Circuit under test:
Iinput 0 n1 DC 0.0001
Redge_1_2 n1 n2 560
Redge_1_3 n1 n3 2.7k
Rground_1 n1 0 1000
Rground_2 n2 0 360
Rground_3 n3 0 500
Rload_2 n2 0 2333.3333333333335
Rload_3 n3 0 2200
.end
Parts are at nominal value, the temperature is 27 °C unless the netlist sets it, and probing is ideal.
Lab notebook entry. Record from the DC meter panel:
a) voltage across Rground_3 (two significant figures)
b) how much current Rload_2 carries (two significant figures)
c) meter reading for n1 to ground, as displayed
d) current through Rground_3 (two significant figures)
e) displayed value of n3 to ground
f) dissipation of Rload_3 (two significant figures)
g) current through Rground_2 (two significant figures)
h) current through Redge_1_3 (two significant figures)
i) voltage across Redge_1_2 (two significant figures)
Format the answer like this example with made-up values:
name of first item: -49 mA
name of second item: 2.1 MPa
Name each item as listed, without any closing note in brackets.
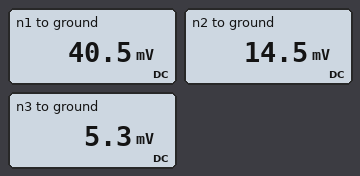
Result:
voltage across Rground_3: 5.3 mV
how much current Rload_2 carries: 6.2 µA
meter reading for n1 to ground, as displayed: 40.5 mV
current through Rground_3: 11 µA
displayed value of n3 to ground: 5.3 mV
dissipation of Rload_3: 13 nW
current through Rground_2: 40 µA
current through Redge_1_3: 13 µA
voltage across Redge_1_2: 26 mV
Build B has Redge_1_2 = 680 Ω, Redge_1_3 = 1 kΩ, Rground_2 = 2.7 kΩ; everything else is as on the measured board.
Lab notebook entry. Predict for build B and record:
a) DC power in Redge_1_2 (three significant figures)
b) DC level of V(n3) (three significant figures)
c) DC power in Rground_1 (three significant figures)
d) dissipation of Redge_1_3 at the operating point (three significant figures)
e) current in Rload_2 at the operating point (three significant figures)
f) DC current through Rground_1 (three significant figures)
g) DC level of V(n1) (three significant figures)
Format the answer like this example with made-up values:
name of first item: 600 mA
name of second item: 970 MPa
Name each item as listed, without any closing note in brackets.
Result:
DC power in Redge_1_2: 367 nW
DC level of V(n3): 13.0 mV
DC power in Rground_1: 2.01 µW
dissipation of Redge_1_3 at the operating point: 1.02 µW
current in Rload_2 at the operating point: 12.5 µA
DC current through Rground_1: 44.9 µA
DC level of V(n1): 44.9 mV
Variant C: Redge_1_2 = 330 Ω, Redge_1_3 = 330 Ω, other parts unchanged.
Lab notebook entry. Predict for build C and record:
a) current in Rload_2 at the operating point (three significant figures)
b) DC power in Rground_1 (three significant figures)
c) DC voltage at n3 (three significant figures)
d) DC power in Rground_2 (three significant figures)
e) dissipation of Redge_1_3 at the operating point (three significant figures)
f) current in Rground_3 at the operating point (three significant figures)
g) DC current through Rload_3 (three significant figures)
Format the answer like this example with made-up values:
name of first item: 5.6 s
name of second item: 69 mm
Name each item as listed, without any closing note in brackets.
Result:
current in Rload_2 at the operating point: 5.32 µA
DC power in Rground_1: 653 nW
DC voltage at n3: 14.1 mV
DC power in Rground_2: 428 nW
dissipation of Redge_1_3 at the operating point: 396 nW
current in Rground_3 at the operating point: 28.2 µA
DC current through Rload_3: 6.42 µA
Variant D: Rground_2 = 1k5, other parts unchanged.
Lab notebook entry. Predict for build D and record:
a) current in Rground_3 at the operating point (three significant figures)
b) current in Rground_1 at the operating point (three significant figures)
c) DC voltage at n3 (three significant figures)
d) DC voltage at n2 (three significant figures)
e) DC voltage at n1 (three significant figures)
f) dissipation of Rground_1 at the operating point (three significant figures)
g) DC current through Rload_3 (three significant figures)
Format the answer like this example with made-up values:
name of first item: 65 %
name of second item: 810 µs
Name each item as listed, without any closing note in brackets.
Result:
current in Rground_3 at the operating point: 13.1 µA
current in Rground_1 at the operating point: 50.0 µA
DC voltage at n3: 6.55 mV
DC voltage at n2: 31.0 mV
DC voltage at n1: 50.0 mV
dissipation of Rground_1 at the operating point: 2.50 µW
DC current through Rload_3: 2.98 µA
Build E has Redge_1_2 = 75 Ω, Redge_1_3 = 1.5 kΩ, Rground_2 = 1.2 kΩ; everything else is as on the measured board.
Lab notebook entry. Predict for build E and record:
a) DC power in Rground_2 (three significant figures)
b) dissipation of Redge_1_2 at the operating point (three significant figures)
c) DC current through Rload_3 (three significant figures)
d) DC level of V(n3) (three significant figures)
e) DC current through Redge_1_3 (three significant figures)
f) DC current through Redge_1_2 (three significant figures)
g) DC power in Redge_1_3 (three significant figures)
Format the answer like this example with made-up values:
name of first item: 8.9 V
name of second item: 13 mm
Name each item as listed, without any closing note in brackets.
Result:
DC power in Rground_2: 970 nW
dissipation of Redge_1_2 at the operating point: 139 nW
DC current through Rload_3: 3.63 µA
DC level of V(n3): 7.98 mV
DC current through Redge_1_3: 19.6 µA
DC current through Redge_1_2: 43.1 µA
DC power in Redge_1_3: 575 nW
